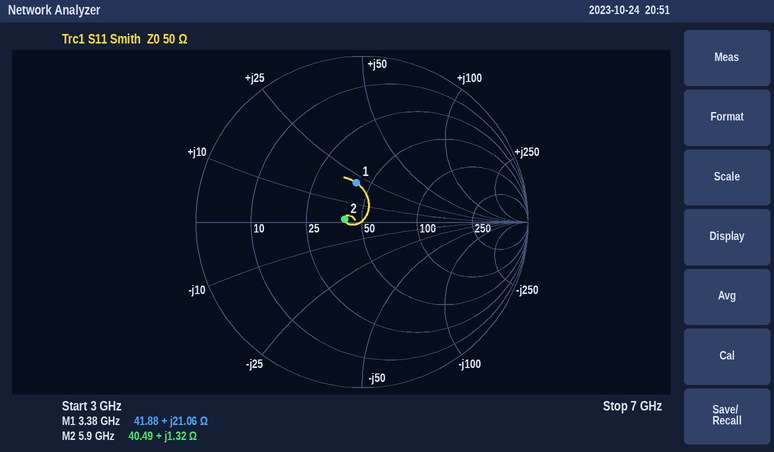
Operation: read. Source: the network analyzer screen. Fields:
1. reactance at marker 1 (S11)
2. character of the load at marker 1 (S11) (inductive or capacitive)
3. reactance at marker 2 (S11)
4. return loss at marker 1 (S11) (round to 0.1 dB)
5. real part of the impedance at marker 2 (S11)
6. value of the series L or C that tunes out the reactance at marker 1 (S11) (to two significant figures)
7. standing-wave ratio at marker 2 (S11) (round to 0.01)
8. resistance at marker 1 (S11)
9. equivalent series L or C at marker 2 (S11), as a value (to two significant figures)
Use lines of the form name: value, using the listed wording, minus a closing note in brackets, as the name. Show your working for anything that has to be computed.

reactance at marker 1: +21.06 Ω
character of the load at marker 1 (S11): inductive
reactance at marker 2: +1.32 Ω
return loss at marker 1 (S11): 12.4 dB
real part of the impedance at marker 2: 40.49 Ω
value of the series L or C that tunes out the reactance at marker 1 (S11): C = 1/(2π × 3.38 GHz × 21.06 Ω) ≈ 2.2 pF
standing-wave ratio at marker 2 (S11): 1.24
resistance at marker 1: 41.88 Ω
equivalent series L or C at marker 2 (S11), as a value: L = 1.32 Ω/(2π × 5.9 GHz) ≈ 36 pH
